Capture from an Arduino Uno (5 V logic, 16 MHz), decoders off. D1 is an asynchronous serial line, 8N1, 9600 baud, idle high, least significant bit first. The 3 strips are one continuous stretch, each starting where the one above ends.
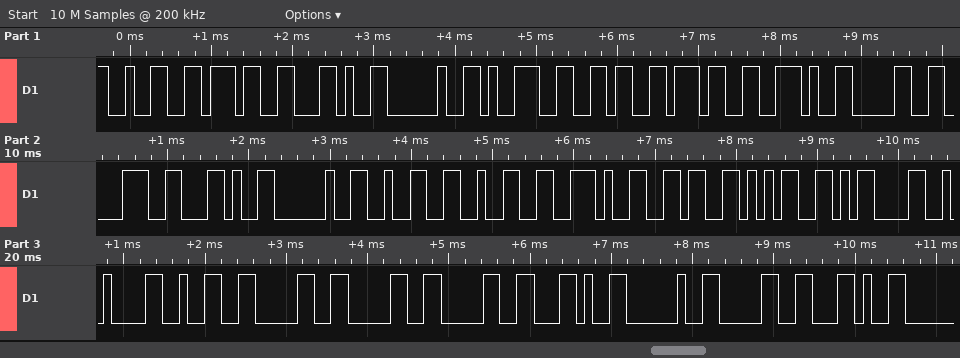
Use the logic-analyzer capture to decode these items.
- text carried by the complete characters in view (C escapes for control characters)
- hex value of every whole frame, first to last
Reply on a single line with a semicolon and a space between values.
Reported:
"27, 967.08, 22.65\r\n2000, 0,"; 32 37 2C 20 39 36 37 2E 30 38 2C 20 32 32 2E 36 35 0D 0A 32 30 30 30 2C 20 30 2C
